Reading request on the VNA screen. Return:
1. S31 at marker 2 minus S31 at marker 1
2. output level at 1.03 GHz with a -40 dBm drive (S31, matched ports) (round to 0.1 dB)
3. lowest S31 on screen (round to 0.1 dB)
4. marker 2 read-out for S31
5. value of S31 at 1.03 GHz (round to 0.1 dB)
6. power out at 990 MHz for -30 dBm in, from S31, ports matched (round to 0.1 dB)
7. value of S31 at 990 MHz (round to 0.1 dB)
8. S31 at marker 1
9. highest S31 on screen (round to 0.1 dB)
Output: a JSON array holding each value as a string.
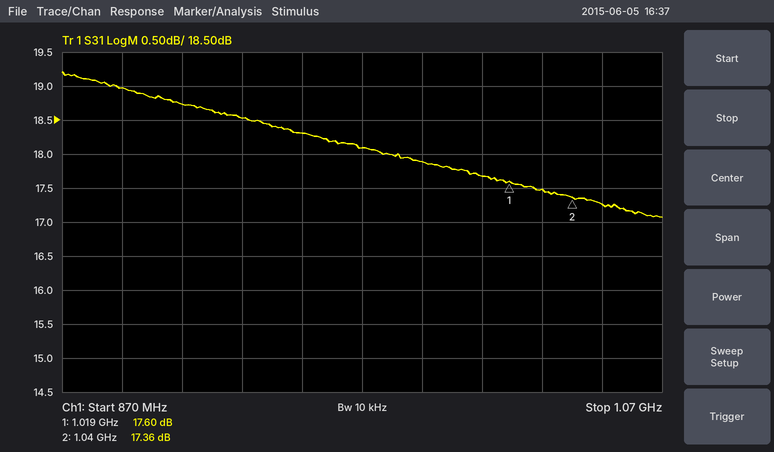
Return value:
["-0.24 dB", "-22.5 dBm", "17.1 dB", "17.36 dB", "17.5 dB", "-12.1 dBm", "17.9 dB", "17.60 dB", "19.2 dB"]
